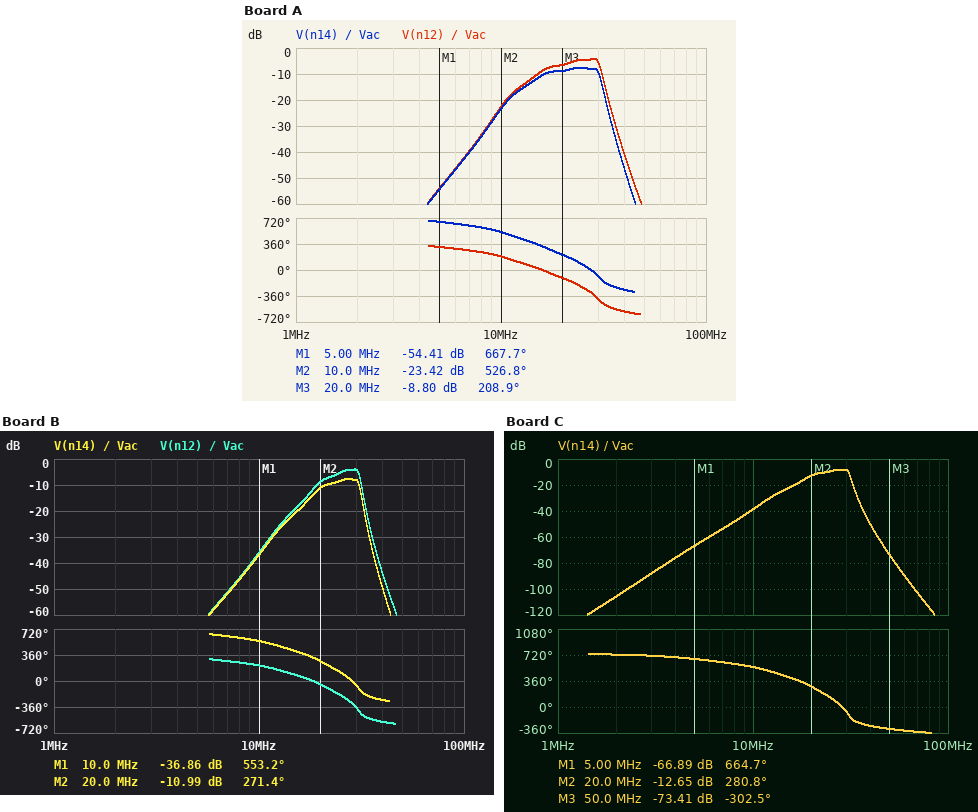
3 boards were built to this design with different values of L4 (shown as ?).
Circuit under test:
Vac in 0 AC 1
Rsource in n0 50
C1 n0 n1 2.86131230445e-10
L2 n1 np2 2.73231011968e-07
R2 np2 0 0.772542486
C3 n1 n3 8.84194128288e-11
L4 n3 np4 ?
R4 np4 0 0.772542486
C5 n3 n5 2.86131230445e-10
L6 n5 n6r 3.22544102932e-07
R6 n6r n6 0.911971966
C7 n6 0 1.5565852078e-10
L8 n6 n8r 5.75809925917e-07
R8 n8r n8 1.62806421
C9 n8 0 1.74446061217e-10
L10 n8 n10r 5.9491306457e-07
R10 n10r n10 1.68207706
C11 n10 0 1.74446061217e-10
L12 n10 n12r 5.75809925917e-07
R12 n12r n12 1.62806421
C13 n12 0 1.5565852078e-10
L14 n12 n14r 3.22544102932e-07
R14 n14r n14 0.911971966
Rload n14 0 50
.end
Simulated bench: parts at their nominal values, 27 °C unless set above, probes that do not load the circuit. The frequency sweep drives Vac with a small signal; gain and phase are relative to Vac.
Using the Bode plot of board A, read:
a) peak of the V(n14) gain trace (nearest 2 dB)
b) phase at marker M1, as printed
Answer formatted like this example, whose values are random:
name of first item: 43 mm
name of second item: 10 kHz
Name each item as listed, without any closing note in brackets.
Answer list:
peak of the V(n14) gain trace: -8 dB
phase at marker M1, as printed: 667.7 deg
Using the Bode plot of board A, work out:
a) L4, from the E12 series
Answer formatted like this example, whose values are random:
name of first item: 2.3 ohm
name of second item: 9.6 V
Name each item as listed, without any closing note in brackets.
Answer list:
L4, from the E12 series: 560 nH
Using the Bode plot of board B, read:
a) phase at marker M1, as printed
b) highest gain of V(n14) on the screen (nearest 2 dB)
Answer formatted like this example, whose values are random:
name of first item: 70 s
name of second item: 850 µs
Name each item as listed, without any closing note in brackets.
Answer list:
phase at marker M1, as printed: 553.2 deg
highest gain of V(n14) on the screen: -8 dB
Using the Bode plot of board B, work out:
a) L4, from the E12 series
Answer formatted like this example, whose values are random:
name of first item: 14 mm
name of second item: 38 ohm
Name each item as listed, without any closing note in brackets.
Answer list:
L4, from the E12 series: 180 nH
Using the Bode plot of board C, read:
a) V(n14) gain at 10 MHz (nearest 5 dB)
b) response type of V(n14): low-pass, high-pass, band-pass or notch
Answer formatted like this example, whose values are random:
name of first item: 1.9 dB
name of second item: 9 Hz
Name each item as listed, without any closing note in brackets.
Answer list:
V(n14) gain at 10 MHz: -40 dB
response type of V(n14): low-pass, high-pass, band-pass or notch: band-pass
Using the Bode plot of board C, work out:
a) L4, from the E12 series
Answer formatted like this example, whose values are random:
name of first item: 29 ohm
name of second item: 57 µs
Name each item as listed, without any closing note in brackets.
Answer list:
L4, from the E12 series: 150 nH
